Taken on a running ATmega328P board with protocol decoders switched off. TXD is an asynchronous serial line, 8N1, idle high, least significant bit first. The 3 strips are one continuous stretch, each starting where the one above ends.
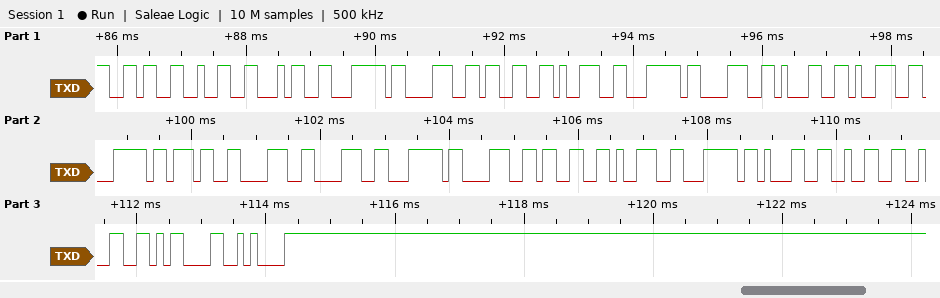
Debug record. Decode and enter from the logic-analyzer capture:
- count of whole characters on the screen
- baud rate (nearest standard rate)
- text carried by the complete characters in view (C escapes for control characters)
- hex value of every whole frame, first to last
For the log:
25
9600 baud
"624|839|819|788|839|122\r\n"
36 32 34 7C 38 33 39 7C 38 31 39 7C 37 38 38 7C 38 33 39 7C 31 32 32 0D 0A
